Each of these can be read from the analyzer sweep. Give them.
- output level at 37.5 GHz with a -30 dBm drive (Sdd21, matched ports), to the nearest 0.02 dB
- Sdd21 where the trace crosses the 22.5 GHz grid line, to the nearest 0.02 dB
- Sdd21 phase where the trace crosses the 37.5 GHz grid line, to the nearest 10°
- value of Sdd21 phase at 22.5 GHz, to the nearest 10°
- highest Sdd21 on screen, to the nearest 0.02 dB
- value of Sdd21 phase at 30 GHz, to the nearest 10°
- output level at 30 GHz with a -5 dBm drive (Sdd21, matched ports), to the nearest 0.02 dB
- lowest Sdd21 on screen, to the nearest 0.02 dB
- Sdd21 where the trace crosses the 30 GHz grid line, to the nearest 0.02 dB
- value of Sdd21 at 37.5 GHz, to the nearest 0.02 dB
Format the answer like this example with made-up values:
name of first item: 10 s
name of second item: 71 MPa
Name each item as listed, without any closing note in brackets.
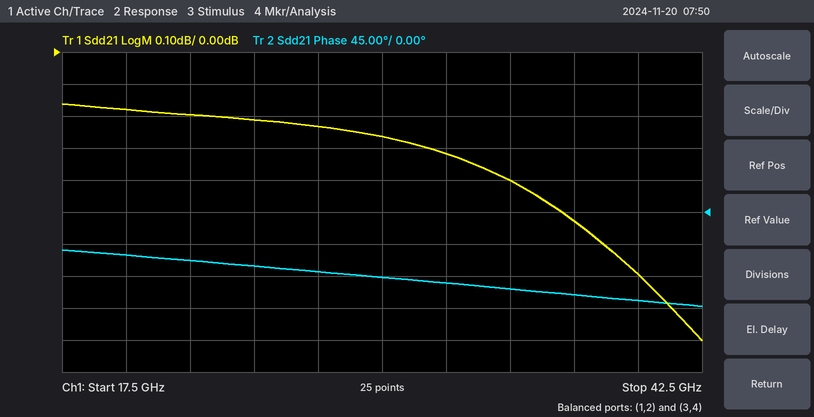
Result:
output level at 37.5 GHz with a -30 dBm drive (Sdd21, matched ports), to the nearest 0.02 dB: -30.52 dBm
Sdd21 where the trace crosses the 22.5 GHz grid line, to the nearest 0.02 dB: -0.20 dB
Sdd21 phase where the trace crosses the 37.5 GHz grid line, to the nearest 10°: -120°
value of Sdd21 phase at 22.5 GHz, to the nearest 10°: -70°
highest Sdd21 on screen, to the nearest 0.02 dB: -0.16 dB
value of Sdd21 phase at 30 GHz, to the nearest 10°: -90°
output level at 30 GHz with a -5 dBm drive (Sdd21, matched ports), to the nearest 0.02 dB: -5.26 dBm
lowest Sdd21 on screen, to the nearest 0.02 dB: -0.90 dB
Sdd21 where the trace crosses the 30 GHz grid line, to the nearest 0.02 dB: -0.26 dB
value of Sdd21 at 37.5 GHz, to the nearest 0.02 dB: -0.52 dB
